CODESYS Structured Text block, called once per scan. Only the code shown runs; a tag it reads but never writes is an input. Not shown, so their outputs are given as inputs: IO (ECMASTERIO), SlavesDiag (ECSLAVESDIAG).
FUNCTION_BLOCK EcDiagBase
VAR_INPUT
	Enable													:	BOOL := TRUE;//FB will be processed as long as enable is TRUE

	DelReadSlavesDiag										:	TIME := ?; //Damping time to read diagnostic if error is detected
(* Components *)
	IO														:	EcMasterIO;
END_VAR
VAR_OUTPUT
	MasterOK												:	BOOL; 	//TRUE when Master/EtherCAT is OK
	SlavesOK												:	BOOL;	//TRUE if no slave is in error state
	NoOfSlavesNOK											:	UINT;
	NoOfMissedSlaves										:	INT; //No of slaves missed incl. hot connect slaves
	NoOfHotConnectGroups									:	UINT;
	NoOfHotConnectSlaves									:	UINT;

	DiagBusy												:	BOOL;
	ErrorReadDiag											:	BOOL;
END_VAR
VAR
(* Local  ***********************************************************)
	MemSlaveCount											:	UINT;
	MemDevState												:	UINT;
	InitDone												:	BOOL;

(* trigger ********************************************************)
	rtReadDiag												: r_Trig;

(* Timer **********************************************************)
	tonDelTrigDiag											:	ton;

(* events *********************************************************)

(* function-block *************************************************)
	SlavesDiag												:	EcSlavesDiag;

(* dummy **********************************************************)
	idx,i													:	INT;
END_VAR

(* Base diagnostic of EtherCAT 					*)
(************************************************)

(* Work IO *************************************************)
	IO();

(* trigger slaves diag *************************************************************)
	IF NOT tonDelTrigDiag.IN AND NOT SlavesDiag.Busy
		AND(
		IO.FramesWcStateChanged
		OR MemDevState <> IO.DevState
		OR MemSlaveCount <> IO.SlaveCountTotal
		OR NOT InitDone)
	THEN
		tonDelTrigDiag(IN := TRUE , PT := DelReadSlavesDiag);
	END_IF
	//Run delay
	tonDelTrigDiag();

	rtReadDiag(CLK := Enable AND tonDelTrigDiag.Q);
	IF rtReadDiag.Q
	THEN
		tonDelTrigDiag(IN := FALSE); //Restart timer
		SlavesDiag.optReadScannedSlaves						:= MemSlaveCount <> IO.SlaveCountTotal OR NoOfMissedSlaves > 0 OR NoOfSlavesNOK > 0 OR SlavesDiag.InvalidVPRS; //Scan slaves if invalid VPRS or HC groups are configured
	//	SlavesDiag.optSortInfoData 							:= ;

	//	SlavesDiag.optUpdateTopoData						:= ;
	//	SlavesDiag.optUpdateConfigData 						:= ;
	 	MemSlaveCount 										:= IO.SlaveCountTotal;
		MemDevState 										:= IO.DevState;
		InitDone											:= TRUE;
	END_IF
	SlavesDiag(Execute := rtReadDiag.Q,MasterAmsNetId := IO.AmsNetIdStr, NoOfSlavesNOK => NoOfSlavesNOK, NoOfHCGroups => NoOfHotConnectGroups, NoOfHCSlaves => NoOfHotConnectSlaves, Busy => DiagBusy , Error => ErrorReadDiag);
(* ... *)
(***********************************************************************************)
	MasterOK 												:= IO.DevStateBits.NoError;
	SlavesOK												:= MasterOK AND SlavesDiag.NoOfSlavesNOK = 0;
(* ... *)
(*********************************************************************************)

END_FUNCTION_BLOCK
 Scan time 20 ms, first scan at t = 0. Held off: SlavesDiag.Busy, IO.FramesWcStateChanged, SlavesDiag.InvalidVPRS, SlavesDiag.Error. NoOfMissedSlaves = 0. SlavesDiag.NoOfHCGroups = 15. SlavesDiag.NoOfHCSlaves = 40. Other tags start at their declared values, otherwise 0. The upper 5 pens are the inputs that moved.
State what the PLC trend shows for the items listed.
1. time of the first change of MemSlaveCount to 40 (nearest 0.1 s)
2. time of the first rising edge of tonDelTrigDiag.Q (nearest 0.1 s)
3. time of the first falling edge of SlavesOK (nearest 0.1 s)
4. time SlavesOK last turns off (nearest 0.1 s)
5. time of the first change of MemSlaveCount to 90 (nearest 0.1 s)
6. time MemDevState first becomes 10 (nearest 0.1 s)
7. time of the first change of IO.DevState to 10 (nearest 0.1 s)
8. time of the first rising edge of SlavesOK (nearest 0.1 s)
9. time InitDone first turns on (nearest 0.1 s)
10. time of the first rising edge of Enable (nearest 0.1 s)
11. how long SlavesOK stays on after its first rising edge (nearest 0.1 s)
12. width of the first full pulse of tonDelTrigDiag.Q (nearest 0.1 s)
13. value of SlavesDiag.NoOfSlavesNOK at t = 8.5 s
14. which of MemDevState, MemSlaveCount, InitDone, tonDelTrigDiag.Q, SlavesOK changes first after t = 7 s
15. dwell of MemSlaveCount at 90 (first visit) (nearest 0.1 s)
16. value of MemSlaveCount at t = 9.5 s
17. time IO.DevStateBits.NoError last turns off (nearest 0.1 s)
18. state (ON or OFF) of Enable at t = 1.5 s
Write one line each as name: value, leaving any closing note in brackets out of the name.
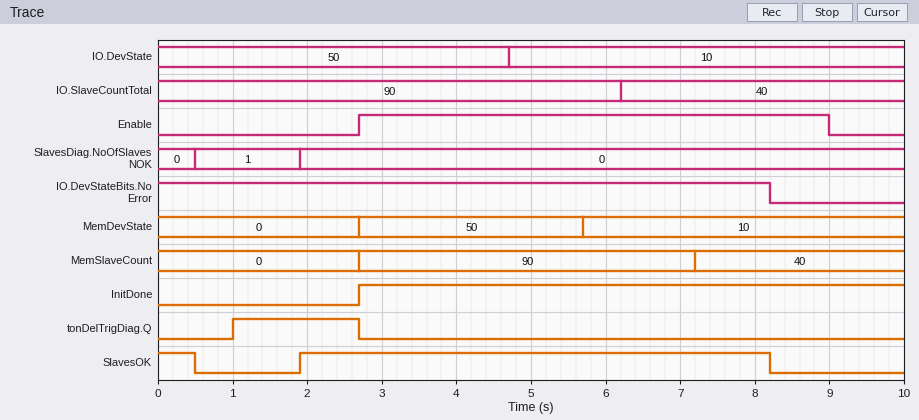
time of the first change of MemSlaveCount to 40: 7.2 s
time of the first rising edge of tonDelTrigDiag.Q: 1.0 s
time of the first falling edge of SlavesOK: 0.5 s
time SlavesOK last turns off: 8.2 s
time of the first change of MemSlaveCount to 90: 2.7 s
time MemDevState first becomes 10: 5.7 s
time of the first change of IO.DevState to 10: 4.7 s
time of the first rising edge of SlavesOK: 1.9 s
time InitDone first turns on: 2.7 s
time of the first rising edge of Enable: 2.7 s
how long SlavesOK stays on after its first rising edge: 6.3 s
width of the first full pulse of tonDelTrigDiag.Q: 1.7 s
value of SlavesDiag.NoOfSlavesNOK at t = 8.5 s: 0
which of MemDevState, MemSlaveCount, InitDone, tonDelTrigDiag.Q, SlavesOK changes first after t = 7 s: MemSlaveCount
dwell of MemSlaveCount at 90 (first visit): 4.5 s
value of MemSlaveCount at t = 9.5 s: 40
time IO.DevStateBits.NoError last turns off: 8.2 s
state (ON or OFF) of Enable at t = 1.5 s: OFF
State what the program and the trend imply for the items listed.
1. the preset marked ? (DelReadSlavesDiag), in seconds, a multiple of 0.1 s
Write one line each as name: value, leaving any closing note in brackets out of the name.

the preset marked ? (DelReadSlavesDiag), in seconds, a multiple of 0.1 s: 1.0 s
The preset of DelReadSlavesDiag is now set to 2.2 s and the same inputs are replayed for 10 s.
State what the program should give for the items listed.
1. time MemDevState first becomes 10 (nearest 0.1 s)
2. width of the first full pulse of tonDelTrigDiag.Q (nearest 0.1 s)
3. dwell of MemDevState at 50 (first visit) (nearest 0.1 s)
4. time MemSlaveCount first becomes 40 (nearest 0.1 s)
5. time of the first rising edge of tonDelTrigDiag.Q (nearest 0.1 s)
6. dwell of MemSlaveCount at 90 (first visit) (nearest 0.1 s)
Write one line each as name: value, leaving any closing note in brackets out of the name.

time MemDevState first becomes 10: 6.9 s
width of the first full pulse of tonDelTrigDiag.Q: 0.5 s
dwell of MemDevState at 50 (first visit): 4.2 s
time MemSlaveCount first becomes 40: 6.9 s
time of the first rising edge of tonDelTrigDiag.Q: 2.2 s
dwell of MemSlaveCount at 90 (first visit): 4.2 s
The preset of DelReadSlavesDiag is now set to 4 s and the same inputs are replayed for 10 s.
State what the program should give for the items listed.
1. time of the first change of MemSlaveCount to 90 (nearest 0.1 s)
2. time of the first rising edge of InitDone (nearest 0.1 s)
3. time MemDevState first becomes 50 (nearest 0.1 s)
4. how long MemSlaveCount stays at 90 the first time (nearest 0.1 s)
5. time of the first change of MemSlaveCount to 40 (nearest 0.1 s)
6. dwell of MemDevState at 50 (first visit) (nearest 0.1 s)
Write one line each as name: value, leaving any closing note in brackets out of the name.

time of the first change of MemSlaveCount to 90: 4.0 s
time of the first rising edge of InitDone: 4.0 s
time MemDevState first becomes 50: 4.0 s
how long MemSlaveCount stays at 90 the first time: 4.7 s
time of the first change of MemSlaveCount to 40: 8.7 s
dwell of MemDevState at 50 (first visit): 4.7 s
